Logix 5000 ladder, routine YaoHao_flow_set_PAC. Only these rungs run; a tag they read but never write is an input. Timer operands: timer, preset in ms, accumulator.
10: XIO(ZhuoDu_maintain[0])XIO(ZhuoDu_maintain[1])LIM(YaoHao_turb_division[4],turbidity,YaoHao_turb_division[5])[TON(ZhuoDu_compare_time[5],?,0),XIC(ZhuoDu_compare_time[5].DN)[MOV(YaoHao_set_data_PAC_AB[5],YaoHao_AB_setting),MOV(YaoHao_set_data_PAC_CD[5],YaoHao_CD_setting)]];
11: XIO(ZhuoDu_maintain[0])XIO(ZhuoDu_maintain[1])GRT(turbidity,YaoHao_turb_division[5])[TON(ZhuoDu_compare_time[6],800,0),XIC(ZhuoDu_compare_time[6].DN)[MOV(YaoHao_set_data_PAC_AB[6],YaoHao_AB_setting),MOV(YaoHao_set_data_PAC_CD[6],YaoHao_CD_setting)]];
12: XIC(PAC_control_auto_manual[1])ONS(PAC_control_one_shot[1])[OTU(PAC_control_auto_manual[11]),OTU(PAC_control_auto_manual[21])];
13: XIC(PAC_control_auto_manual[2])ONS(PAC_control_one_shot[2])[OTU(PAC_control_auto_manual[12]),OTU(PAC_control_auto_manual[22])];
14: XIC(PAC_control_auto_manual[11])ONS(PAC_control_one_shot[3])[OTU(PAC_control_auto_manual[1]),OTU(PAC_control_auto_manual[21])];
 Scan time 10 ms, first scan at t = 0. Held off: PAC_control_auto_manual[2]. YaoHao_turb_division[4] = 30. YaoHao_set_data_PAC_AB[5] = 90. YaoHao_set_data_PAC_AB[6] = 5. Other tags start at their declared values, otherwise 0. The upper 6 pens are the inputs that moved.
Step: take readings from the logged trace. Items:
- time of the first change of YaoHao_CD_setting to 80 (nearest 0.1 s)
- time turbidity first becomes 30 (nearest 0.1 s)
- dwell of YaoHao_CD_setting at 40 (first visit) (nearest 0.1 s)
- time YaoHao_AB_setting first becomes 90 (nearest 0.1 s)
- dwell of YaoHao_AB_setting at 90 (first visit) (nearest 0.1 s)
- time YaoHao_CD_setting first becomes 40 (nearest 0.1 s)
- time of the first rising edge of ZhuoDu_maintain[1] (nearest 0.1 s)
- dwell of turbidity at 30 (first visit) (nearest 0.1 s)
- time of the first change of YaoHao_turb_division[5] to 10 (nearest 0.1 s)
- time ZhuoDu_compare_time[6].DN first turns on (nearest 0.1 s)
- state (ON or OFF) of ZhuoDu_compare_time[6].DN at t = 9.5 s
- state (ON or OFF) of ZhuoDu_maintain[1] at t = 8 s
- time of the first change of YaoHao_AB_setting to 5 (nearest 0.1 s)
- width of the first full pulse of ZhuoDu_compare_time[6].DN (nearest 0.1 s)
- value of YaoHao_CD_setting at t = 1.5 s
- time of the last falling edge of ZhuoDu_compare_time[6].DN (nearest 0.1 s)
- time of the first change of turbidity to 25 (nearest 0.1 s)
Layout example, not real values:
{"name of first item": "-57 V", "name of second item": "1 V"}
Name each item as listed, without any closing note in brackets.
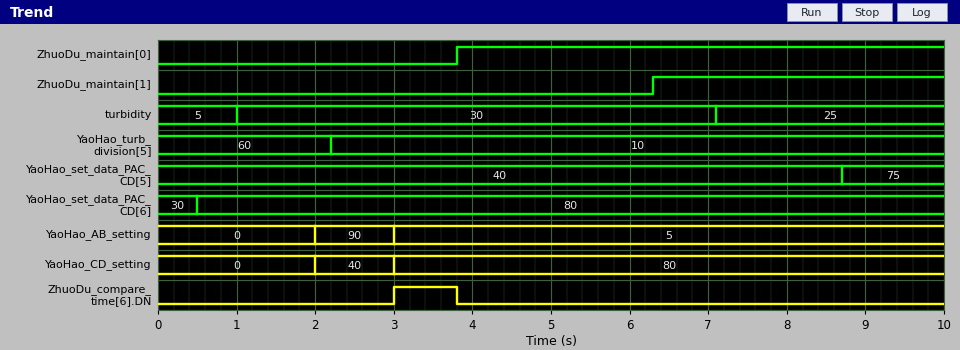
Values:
{"time of the first change of YaoHao_CD_setting to 80": "3.0 s", "time turbidity first becomes 30": "1.0 s", "dwell of YaoHao_CD_setting at 40 (first visit)": "1.0 s", "time YaoHao_AB_setting first becomes 90": "2.0 s", "dwell of YaoHao_AB_setting at 90 (first visit)": "1.0 s", "time YaoHao_CD_setting first becomes 40": "2.0 s", "time of the first rising edge of ZhuoDu_maintain[1]": "6.3 s", "dwell of turbidity at 30 (first visit)": "6.1 s", "time of the first change of YaoHao_turb_division[5] to 10": "2.2 s", "time ZhuoDu_compare_time[6].DN first turns on": "3.0 s", "state (ON or OFF) of ZhuoDu_compare_time[6].DN at t = 9.5 s": "OFF", "state (ON or OFF) of ZhuoDu_maintain[1] at t = 8 s": "ON", "time of the first change of YaoHao_AB_setting to 5": "3.0 s", "width of the first full pulse of ZhuoDu_compare_time[6].DN": "0.8 s", "value of YaoHao_CD_setting at t = 1.5 s": "0", "time of the last falling edge of ZhuoDu_compare_time[6].DN": "3.8 s", "time of the first change of turbidity to 25": "7.1 s"}
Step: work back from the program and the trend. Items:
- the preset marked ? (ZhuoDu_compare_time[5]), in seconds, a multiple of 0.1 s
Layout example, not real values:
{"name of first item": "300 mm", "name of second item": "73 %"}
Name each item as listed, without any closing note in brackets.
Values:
{"the preset marked ? (ZhuoDu_compare_time[5]), in seconds, a multiple of 0.1 s": "1.0 s"}
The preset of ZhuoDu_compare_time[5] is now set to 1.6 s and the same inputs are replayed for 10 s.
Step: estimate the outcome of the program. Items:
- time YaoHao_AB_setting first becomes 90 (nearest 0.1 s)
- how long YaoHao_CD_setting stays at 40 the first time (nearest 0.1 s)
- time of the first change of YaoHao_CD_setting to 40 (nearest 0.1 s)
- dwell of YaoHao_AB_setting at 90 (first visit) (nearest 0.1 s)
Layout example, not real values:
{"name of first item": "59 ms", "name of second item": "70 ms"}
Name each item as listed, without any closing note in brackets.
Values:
{"time YaoHao_AB_setting first becomes 90": "2.6 s", "how long YaoHao_CD_setting stays at 40 the first time": "0.4 s", "time of the first change of YaoHao_CD_setting to 40": "2.6 s", "dwell of YaoHao_AB_setting at 90 (first visit)": "0.4 s"}
